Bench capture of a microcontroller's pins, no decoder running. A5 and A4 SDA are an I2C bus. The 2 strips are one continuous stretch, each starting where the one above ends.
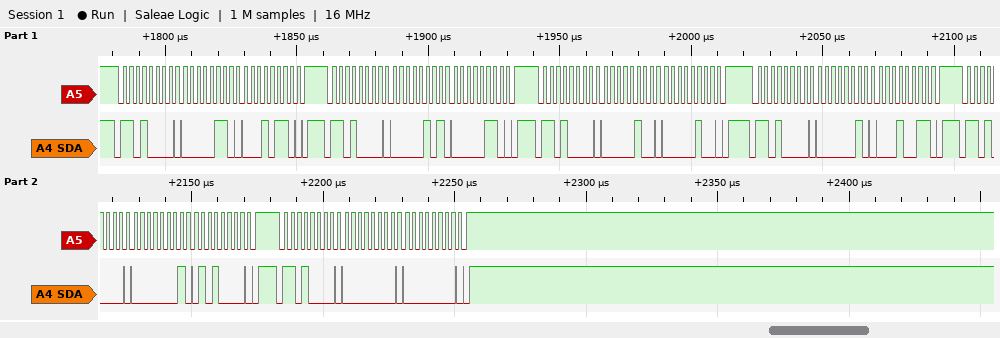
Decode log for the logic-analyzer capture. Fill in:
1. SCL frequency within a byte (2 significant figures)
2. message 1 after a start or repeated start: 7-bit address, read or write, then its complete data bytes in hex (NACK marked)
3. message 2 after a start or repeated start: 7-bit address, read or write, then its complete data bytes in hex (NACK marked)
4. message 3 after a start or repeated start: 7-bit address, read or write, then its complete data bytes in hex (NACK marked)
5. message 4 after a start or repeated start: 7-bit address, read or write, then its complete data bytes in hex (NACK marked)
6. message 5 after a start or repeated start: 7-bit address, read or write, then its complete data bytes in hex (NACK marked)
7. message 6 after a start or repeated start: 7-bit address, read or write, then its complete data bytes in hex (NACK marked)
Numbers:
400 kHz
0x68 write: 06 16
0x68 write: 05 06
0x68 write: 04 04
0x68 write: 02 13
0x68 write: 01 50
0x68 write: 00 00
